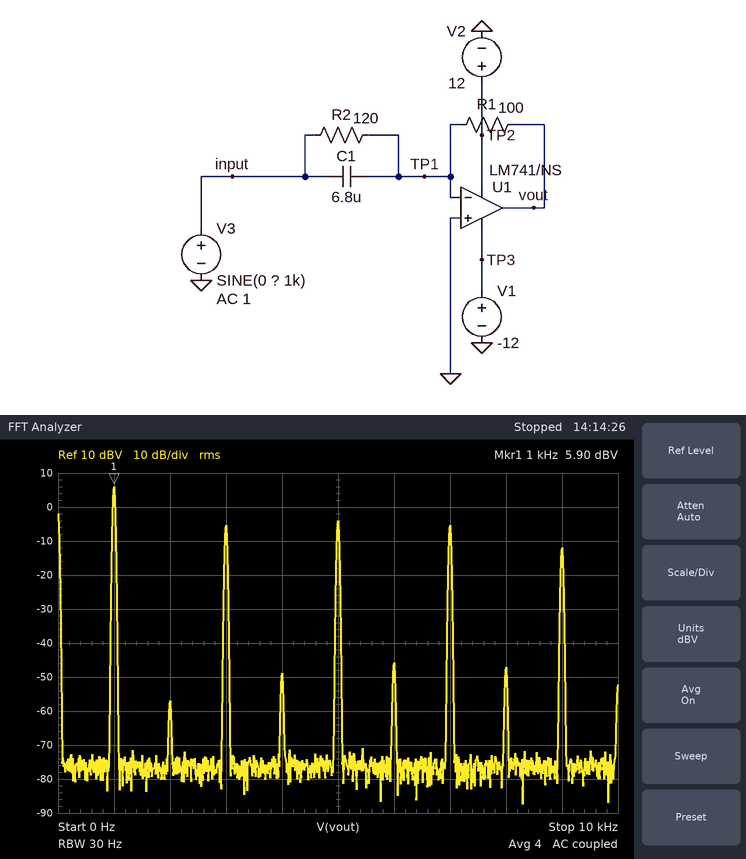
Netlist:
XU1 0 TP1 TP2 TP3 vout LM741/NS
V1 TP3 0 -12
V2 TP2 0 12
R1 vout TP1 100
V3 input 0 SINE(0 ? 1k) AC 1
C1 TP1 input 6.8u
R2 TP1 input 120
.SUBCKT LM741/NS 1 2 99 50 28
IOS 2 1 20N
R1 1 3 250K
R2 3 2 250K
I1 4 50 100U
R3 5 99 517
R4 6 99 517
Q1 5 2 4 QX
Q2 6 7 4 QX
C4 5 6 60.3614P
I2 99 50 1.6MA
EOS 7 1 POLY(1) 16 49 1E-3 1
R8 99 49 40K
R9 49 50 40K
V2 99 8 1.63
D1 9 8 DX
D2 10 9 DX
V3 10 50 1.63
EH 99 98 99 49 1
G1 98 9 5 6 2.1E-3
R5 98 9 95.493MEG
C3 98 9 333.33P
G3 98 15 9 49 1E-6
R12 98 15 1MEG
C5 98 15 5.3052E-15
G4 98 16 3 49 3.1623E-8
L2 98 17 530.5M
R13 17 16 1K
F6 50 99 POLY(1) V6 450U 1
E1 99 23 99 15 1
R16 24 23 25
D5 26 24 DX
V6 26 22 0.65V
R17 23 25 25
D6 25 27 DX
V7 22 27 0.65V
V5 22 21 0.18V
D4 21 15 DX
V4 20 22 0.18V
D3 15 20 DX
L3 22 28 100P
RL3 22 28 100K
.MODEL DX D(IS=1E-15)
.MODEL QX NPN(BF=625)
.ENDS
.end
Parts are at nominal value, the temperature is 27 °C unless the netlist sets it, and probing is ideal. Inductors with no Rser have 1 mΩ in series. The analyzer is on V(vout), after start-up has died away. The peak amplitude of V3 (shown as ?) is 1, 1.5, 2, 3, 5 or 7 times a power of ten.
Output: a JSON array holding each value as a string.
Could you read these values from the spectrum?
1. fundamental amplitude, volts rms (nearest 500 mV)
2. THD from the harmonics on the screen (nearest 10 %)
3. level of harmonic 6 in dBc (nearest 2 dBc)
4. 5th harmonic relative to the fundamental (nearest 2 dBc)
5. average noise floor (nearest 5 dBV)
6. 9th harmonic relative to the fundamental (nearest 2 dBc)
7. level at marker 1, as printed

["2.0 V", "50 %", "-52 dBc", "-10 dBc", "-75 dBV", "-18 dBc", "5.90 dBV"]
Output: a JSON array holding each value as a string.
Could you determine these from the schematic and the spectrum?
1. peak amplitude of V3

["700 mV"]
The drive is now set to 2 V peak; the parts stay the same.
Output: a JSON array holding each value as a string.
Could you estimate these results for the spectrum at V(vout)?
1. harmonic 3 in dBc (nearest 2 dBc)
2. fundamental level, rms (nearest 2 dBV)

["-2 dBc", "0 dBV"]
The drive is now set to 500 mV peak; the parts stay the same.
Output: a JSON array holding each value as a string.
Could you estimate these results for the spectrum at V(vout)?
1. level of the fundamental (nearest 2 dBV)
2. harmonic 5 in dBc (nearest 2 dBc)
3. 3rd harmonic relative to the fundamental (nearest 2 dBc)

["4 dBV", "-44 dBc", "-56 dBc"]
